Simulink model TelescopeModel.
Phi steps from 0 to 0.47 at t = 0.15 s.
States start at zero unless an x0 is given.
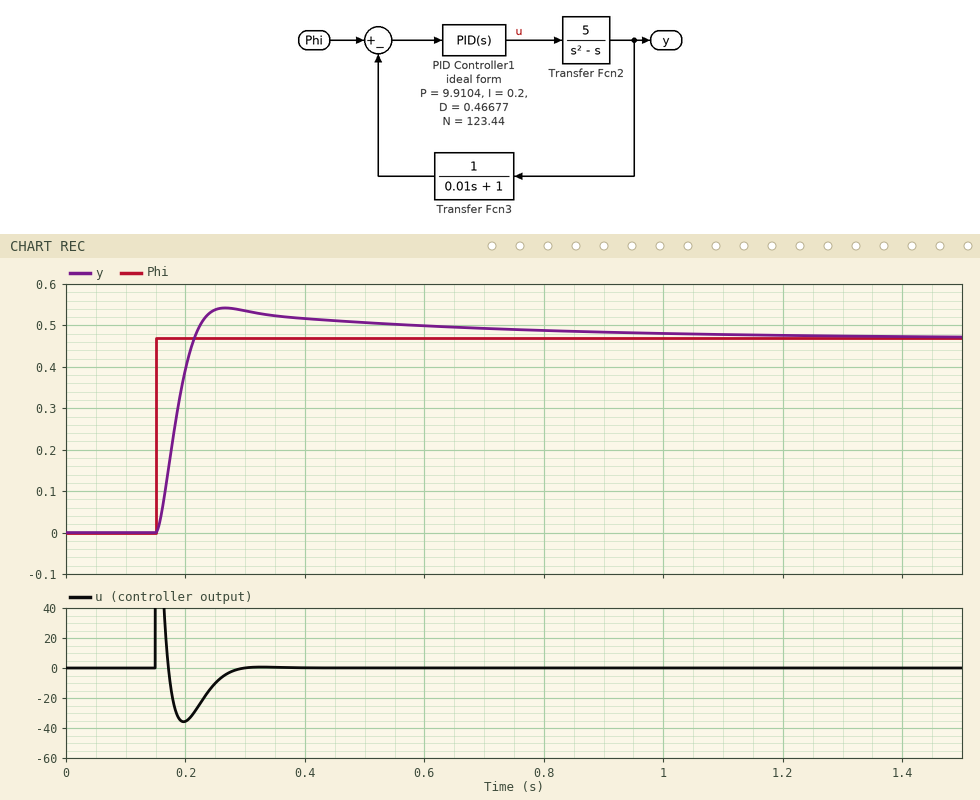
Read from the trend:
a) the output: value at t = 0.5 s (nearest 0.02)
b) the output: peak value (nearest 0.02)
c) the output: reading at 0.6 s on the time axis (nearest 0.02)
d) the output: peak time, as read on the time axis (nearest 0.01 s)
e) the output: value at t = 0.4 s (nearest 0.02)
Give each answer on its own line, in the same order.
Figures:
0.50
0.54
0.50
0.27 s
0.52
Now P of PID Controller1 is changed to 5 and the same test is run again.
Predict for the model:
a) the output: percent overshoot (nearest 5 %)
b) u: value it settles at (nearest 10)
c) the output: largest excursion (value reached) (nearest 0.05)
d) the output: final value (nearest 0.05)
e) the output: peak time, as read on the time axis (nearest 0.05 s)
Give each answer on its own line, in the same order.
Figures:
20 %
0
0.55
0.45
0.45 s
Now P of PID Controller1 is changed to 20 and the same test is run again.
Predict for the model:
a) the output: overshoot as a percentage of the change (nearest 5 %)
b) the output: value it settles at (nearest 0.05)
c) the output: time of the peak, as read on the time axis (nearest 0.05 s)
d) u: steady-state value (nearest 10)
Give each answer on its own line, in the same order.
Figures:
35 %
0.45
0.20 s
0
